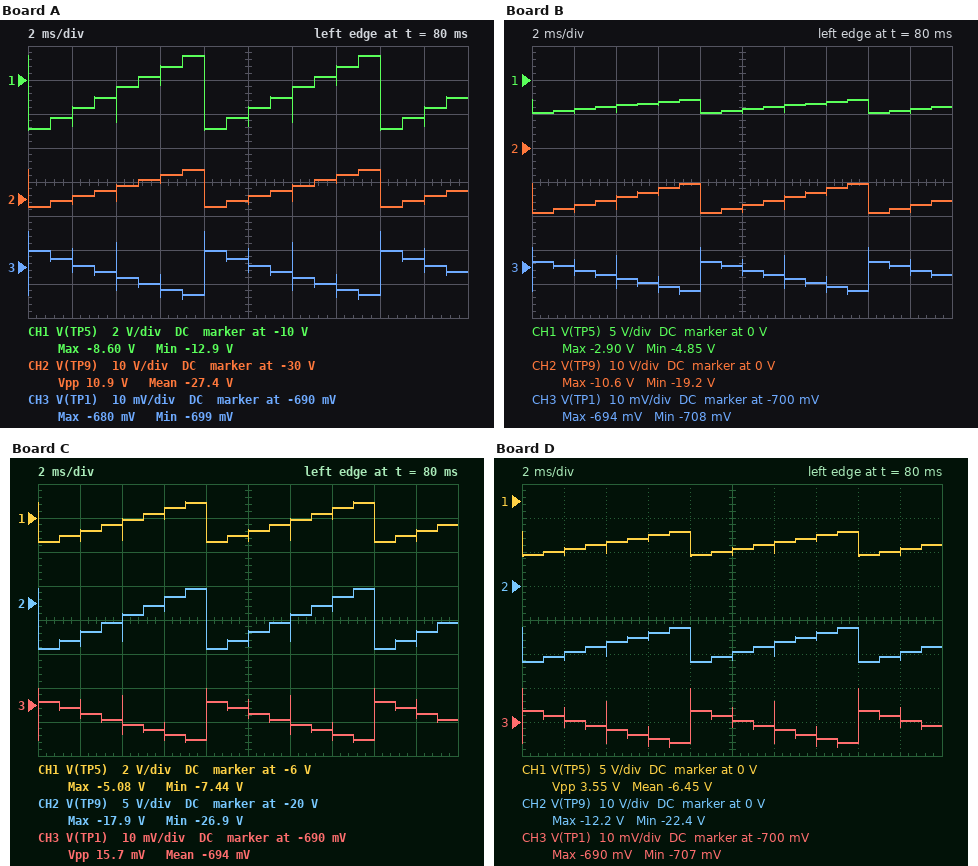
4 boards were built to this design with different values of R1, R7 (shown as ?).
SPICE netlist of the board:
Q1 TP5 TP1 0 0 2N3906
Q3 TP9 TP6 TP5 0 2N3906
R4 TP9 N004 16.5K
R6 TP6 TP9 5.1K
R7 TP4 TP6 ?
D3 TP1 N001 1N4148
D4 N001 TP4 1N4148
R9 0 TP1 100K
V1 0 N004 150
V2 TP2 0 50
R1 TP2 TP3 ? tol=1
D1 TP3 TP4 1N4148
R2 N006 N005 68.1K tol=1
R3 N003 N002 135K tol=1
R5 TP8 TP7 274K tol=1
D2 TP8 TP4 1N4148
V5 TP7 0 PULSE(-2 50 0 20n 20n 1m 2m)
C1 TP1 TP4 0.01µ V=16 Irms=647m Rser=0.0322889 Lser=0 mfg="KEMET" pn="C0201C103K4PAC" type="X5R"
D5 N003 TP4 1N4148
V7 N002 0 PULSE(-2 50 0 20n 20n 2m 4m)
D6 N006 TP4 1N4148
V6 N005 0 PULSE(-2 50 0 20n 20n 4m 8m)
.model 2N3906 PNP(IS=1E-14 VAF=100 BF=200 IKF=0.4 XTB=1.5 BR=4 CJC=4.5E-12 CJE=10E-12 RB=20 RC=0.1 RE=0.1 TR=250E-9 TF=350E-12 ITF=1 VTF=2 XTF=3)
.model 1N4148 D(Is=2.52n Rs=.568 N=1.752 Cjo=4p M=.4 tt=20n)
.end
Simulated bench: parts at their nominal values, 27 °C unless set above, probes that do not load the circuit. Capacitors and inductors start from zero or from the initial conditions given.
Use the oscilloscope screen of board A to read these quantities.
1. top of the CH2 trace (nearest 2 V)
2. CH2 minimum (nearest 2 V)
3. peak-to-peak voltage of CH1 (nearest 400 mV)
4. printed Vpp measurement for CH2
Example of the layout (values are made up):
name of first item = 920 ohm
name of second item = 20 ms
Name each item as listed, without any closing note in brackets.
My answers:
top of the CH2 trace = -22 V
CH2 minimum = -32 V
peak-to-peak voltage of CH1 = 4.4 V
printed Vpp measurement for CH2 = 10.9 V
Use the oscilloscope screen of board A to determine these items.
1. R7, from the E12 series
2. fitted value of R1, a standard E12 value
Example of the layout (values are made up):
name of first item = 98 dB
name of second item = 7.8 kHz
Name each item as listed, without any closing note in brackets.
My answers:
R7, from the E12 series = 3.3 kΩ
fitted value of R1, a standard E12 value = 22 kΩ
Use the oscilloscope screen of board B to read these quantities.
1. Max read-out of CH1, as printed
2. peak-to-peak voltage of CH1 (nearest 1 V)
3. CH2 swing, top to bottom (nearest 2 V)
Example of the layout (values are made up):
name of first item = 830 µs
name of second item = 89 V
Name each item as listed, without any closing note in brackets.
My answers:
Max read-out of CH1, as printed = -2.90 V
peak-to-peak voltage of CH1 = 2 V
CH2 swing, top to bottom = 8 V
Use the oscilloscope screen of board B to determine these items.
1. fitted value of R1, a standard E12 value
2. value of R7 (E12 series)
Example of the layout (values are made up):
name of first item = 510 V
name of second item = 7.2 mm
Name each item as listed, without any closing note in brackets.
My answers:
fitted value of R1, a standard E12 value = 39 kΩ
value of R7 = 1.5 kΩ
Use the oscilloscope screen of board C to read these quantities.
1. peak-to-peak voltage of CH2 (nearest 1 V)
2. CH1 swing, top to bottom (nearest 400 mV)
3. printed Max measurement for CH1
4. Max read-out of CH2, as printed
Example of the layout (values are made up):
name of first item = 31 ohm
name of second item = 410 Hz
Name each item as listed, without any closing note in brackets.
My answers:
peak-to-peak voltage of CH2 = 9 V
CH1 swing, top to bottom = 2.4 V
printed Max measurement for CH1 = -5.08 V
Max read-out of CH2, as printed = -17.9 V
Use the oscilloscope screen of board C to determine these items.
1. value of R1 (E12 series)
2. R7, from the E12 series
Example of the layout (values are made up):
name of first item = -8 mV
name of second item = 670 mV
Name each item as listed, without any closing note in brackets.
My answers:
value of R1 = 22 kΩ
R7, from the E12 series = 1.8 kΩ
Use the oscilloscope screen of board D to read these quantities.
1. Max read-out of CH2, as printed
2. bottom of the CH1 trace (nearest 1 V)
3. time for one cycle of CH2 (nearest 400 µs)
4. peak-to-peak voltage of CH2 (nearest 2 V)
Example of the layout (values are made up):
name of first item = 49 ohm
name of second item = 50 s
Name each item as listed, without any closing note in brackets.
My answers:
Max read-out of CH2, as printed = -12.2 V
bottom of the CH1 trace = -8 V
time for one cycle of CH2 = 8.0 ms
peak-to-peak voltage of CH2 = 10 V
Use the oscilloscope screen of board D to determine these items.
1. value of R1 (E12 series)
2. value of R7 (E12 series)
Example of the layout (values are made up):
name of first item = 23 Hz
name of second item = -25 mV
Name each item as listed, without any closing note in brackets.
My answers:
value of R1 = 39 kΩ
value of R7 = 2.7 kΩ
